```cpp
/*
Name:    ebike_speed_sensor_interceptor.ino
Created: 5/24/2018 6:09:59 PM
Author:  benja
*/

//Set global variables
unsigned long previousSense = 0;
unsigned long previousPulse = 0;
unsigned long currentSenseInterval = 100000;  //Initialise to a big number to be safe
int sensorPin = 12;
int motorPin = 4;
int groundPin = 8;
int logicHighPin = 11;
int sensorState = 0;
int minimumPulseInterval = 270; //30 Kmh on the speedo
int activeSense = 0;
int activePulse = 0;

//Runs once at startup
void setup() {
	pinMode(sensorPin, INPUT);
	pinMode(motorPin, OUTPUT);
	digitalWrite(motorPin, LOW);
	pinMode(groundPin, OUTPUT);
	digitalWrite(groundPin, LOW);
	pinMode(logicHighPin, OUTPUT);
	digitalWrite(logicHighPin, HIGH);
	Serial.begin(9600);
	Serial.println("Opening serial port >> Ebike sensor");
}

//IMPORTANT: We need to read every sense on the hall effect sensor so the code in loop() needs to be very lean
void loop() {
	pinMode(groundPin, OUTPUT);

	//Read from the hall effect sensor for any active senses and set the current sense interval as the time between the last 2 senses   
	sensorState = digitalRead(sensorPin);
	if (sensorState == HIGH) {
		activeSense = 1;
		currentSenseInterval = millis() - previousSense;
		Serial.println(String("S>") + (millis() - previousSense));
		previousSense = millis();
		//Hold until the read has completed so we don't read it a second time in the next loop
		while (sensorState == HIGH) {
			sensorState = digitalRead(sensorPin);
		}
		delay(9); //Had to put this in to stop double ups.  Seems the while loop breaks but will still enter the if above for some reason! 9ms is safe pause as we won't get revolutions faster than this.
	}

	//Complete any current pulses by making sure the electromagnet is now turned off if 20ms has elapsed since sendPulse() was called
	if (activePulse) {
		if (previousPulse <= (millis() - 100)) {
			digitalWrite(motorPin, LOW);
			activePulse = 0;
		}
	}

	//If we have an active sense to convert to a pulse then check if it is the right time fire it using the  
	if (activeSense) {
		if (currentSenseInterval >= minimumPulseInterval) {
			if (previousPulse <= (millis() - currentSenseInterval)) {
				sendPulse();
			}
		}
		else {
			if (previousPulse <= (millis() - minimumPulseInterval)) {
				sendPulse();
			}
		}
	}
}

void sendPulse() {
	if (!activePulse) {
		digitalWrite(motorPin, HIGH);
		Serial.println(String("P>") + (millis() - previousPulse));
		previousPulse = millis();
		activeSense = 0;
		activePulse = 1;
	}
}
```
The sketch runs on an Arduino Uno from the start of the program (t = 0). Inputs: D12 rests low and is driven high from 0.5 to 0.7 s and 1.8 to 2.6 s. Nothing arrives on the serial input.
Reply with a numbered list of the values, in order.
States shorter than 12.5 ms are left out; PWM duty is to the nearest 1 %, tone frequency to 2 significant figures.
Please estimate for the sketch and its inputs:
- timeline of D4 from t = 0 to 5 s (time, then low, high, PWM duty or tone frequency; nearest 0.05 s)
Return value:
1. 0 s low; 0.7 s high; 0.8 s low; 2.6 s high; 2.7 s low
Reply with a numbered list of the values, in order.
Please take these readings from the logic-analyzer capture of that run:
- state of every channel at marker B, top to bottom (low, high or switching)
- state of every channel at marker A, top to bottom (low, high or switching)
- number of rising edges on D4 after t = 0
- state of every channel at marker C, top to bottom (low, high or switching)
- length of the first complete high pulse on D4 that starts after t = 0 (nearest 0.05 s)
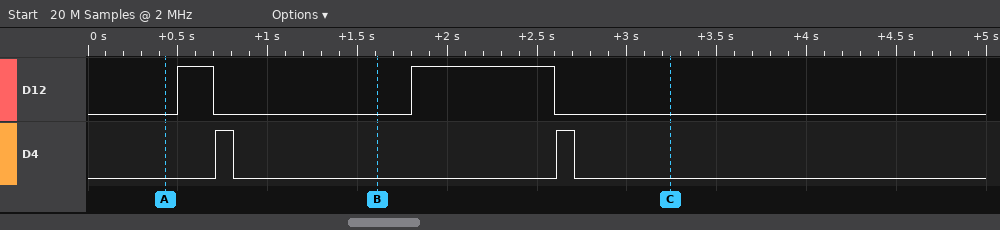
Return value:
1. D12 low, D4 low
2. D12 low, D4 low
3. 2
4. D12 low, D4 low
5. 0.10 s
